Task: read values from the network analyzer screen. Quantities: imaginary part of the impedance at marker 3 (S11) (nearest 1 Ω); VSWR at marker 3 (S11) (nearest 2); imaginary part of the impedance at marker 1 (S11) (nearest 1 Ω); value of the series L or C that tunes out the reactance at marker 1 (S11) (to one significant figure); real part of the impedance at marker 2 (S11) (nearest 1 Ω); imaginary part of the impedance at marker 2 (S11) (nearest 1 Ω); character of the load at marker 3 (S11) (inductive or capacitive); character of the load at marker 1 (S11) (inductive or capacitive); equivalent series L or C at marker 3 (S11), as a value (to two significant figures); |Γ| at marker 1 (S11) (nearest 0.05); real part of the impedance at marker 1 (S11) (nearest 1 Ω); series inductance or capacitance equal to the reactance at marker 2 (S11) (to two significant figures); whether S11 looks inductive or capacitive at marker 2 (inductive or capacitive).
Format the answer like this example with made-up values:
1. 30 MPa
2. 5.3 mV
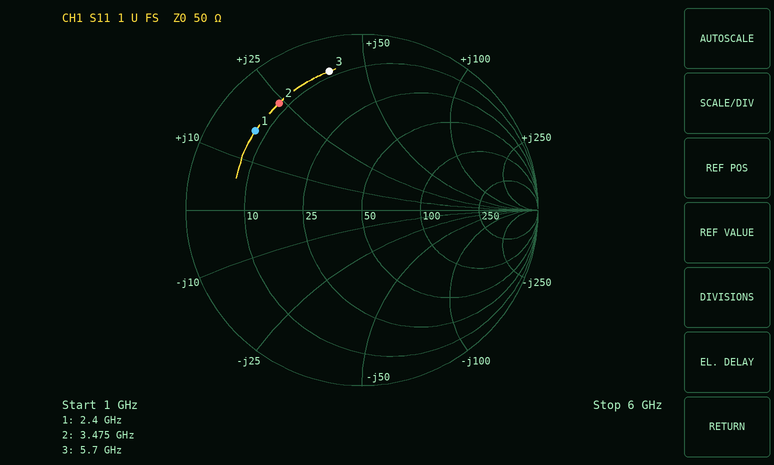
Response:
1. +39 Ω
2. 10
3. +16 Ω
4. 4 pF
5. 8 Ω
6. +24 Ω
7. inductive
8. inductive
9. 1.1 nH
10. 0.75
11. 8 Ω
12. 1.1 nH
13. inductive
